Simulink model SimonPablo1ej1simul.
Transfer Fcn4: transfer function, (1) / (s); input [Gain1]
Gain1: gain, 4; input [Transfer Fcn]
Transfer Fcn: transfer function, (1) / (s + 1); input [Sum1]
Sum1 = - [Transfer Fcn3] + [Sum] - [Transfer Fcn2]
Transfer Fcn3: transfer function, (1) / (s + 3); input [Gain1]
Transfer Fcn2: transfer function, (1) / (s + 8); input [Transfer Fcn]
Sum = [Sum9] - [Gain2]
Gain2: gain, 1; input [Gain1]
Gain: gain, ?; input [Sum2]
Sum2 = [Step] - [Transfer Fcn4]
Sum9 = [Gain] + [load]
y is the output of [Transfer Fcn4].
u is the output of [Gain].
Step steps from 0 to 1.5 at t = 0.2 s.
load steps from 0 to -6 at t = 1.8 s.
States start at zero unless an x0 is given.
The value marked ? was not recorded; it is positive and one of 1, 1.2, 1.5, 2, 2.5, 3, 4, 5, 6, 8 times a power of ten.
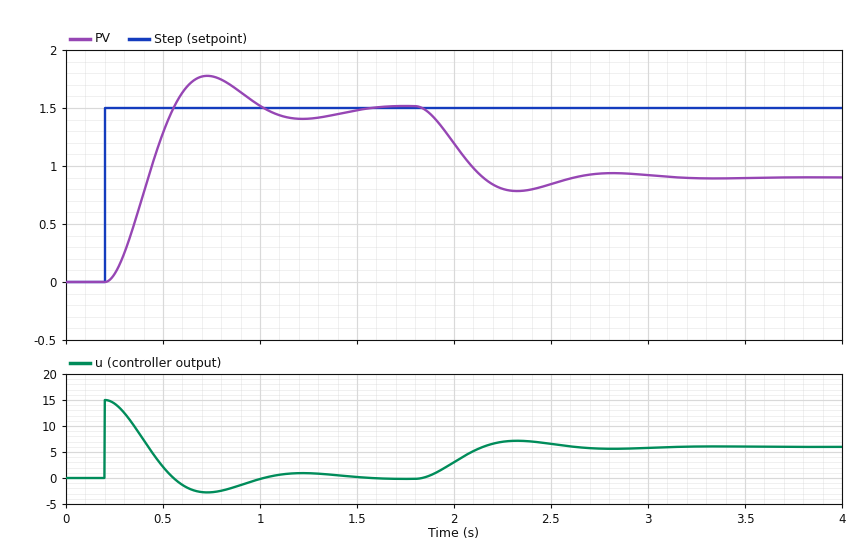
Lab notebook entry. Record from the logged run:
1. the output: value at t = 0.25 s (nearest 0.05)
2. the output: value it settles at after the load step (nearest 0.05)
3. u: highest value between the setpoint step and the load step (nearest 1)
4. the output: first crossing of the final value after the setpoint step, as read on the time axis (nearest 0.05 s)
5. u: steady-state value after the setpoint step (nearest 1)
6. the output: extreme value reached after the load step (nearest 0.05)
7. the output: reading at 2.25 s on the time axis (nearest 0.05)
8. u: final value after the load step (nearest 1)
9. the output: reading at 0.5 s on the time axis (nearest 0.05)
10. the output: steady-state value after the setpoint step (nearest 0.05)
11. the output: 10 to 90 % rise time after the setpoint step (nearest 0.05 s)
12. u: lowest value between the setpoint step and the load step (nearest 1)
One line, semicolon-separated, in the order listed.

0.05; 0.90; 15; 0.55 s; 0; 0.80; 0.80; 6; 1.30; 1.50; 0.25 s; -3
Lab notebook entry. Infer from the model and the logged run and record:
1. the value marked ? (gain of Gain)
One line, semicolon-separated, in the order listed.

10
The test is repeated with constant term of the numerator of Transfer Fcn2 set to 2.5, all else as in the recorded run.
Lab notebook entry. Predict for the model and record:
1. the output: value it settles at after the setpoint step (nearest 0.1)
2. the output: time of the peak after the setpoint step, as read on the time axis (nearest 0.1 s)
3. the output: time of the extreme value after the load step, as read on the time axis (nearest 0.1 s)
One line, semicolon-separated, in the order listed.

1.5; 0.7 s; 2.3 s
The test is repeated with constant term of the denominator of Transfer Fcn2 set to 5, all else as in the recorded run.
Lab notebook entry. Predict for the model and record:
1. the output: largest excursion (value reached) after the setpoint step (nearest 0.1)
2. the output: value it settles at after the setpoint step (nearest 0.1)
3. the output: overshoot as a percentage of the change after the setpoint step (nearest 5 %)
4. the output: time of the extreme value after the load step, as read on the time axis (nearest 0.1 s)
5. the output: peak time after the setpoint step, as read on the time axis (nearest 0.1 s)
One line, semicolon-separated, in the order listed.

1.8; 1.5; 20 %; 2.3 s; 0.7 s
